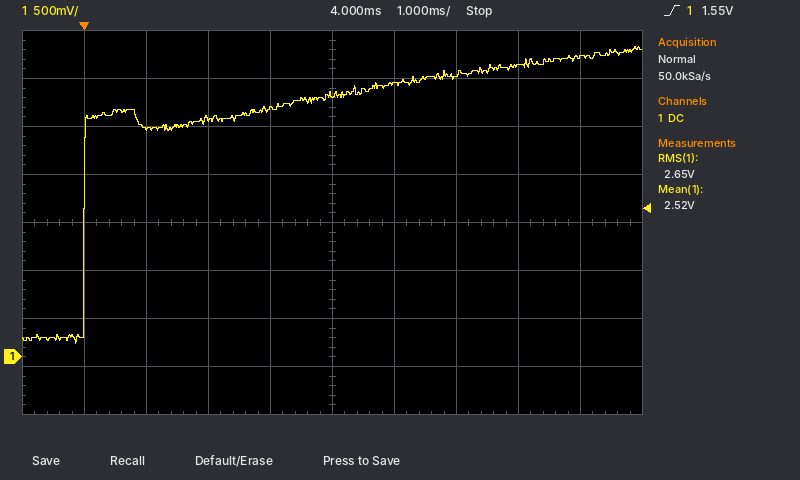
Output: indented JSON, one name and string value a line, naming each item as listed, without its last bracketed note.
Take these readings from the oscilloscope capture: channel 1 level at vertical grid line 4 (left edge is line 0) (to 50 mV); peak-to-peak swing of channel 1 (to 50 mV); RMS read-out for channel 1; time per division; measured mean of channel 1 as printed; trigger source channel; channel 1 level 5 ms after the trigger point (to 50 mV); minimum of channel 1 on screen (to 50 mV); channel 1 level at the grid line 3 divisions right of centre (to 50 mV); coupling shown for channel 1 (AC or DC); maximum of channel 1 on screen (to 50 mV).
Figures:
{
  "channel 1 level at vertical grid line 4 (left edge is line 0)": "2.60 V",
  "peak-to-peak swing of channel 1": "3.10 V",
  "RMS read-out for channel 1": "2.65 V",
  "time per division": "1 ms",
  "measured mean of channel 1 as printed": "2.52 V",
  "trigger source channel": "channel 1",
  "channel 1 level 5 ms after the trigger point": "2.85 V",
  "minimum of channel 1 on screen": "150 mV",
  "channel 1 level at the grid line 3 divisions right of centre": "3.05 V",
  "coupling shown for channel 1": "DC",
  "maximum of channel 1 on screen": "3.25 V"
}
